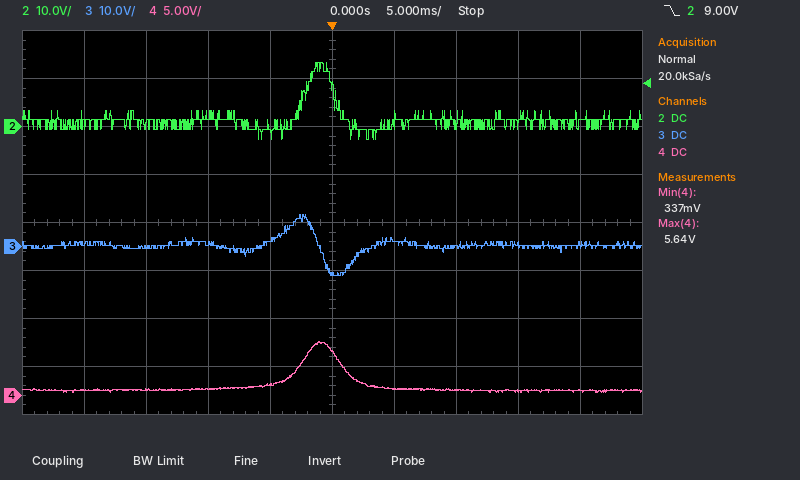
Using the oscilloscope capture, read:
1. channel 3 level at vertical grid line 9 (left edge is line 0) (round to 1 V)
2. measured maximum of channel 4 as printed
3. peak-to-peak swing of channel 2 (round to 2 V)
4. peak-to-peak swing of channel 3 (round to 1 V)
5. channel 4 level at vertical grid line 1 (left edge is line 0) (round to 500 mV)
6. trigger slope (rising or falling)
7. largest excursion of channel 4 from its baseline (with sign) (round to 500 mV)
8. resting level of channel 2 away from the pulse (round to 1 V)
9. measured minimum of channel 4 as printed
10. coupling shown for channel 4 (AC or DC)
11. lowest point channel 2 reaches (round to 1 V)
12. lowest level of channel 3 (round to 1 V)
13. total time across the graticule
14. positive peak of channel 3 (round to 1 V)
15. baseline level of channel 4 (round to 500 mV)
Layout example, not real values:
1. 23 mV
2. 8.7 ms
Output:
1. 0 V
2. 5.64 V
3. 16 V
4. 13 V
5. 500 mV
6. falling
7. +5.0 V
8. 1 V
9. 337 mV
10. DC
11. -3 V
12. -6 V
13. 50 ms
14. 7 V
15. 500 mV
